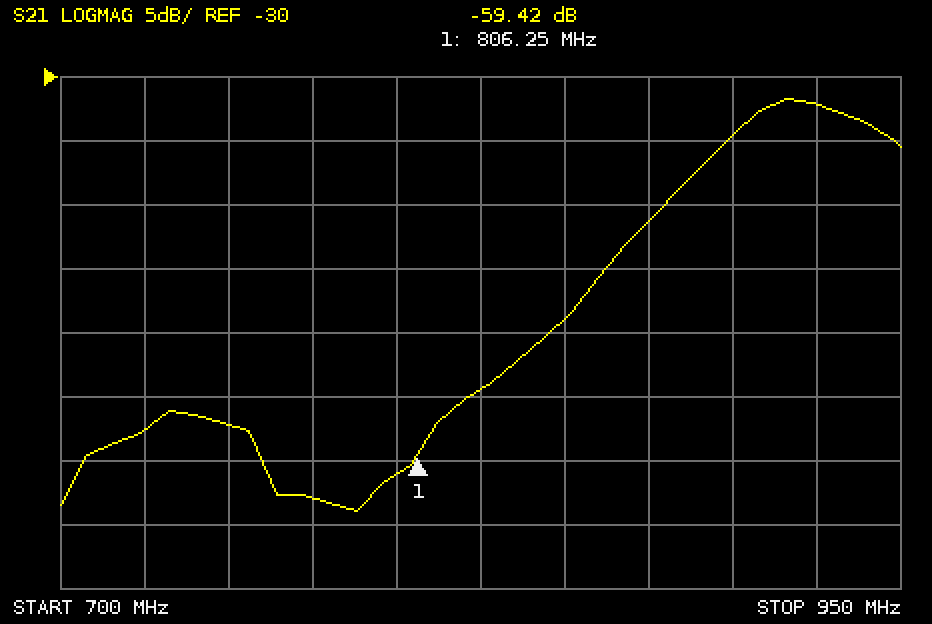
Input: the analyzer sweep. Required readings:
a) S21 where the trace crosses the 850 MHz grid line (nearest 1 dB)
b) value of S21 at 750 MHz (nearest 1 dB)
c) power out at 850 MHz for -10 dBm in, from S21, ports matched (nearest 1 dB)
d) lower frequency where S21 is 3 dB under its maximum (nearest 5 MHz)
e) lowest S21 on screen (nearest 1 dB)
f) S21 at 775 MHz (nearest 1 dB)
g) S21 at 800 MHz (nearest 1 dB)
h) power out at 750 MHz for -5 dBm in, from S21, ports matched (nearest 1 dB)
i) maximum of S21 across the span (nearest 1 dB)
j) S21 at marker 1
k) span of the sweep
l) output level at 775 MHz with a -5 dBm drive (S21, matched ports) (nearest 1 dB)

-49 dB
-57 dB
-59 dBm
900 MHz
-64 dB
-63 dB
-61 dB
-62 dBm
-32 dB
-59.42 dB
250 MHz
-68 dBm
